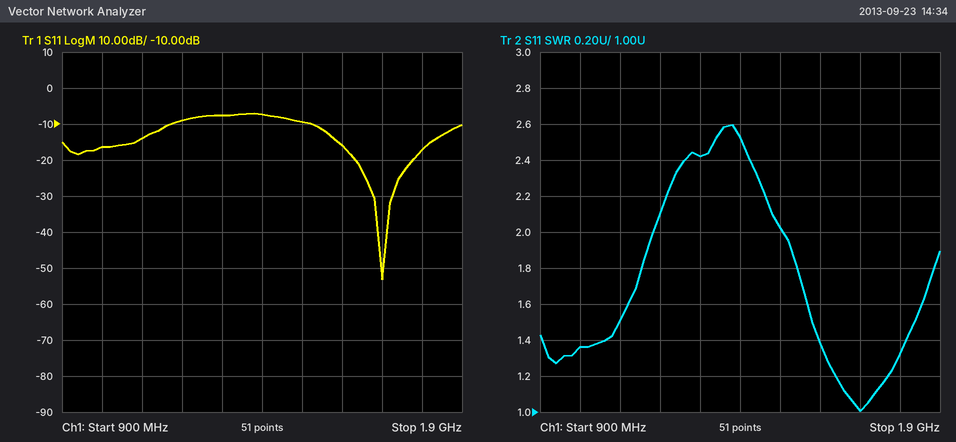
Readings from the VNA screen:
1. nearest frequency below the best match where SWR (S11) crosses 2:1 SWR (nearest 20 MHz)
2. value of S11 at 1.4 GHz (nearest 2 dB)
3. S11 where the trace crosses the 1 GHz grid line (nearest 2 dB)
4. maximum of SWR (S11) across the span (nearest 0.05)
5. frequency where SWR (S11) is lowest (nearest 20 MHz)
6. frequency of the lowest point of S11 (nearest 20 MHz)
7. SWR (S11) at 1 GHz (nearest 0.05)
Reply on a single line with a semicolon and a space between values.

1.50 GHz; -8 dB; -16 dB; 2.60; 1.70 GHz; 1.70 GHz; 1.35
